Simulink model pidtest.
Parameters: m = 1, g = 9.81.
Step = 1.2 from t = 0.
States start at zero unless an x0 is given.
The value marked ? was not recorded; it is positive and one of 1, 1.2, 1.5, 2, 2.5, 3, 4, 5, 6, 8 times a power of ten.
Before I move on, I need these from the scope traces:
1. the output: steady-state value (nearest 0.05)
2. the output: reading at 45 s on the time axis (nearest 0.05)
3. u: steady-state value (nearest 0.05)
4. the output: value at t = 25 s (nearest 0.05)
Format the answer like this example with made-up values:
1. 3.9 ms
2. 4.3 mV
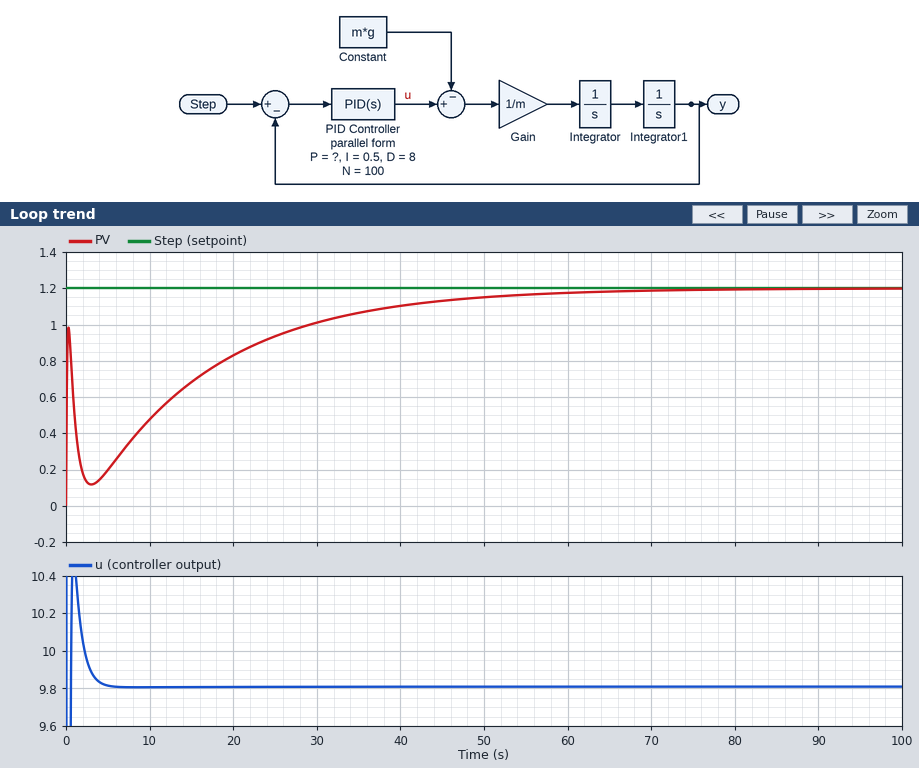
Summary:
1. 1.20
2. 1.15
3. 9.80
4. 0.95
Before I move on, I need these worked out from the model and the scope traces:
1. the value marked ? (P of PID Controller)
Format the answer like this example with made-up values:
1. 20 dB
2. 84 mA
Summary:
1. 8
